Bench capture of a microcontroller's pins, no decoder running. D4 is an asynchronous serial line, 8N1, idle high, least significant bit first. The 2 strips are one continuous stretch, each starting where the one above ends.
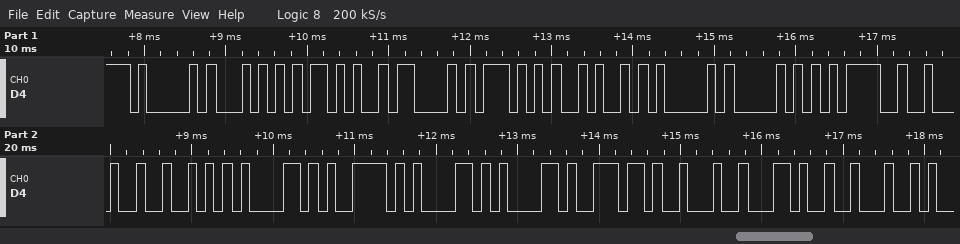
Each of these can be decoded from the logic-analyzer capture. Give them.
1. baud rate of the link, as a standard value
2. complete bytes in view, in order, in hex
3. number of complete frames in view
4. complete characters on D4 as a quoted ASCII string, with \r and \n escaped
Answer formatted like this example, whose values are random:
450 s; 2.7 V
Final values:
9600 baud; 41 54 2B 43 57 4A 41 50 3D 22 52 61 79 61 61 6E 22 2C 22; 19; "AT+CWJAP=\"Rayaan\",\""
